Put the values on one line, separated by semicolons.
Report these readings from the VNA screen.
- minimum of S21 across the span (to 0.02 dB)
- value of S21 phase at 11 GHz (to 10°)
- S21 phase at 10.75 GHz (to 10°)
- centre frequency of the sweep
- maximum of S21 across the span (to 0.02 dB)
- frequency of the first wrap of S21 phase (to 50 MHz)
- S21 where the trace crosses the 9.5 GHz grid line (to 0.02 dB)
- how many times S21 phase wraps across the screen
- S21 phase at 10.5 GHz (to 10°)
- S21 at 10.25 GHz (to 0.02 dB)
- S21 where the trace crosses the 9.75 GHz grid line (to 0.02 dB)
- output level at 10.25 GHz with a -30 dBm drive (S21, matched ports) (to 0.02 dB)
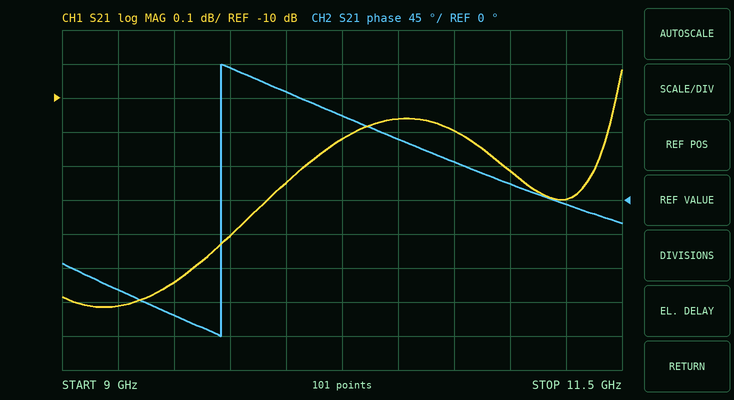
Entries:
-10.62 dB; 20°; 50°; 10.25 GHz; -9.92 dB; 9.70 GHz; -10.54 dB; 1; 80°; -10.12 dB; -10.40 dB; -40.12 dBm
